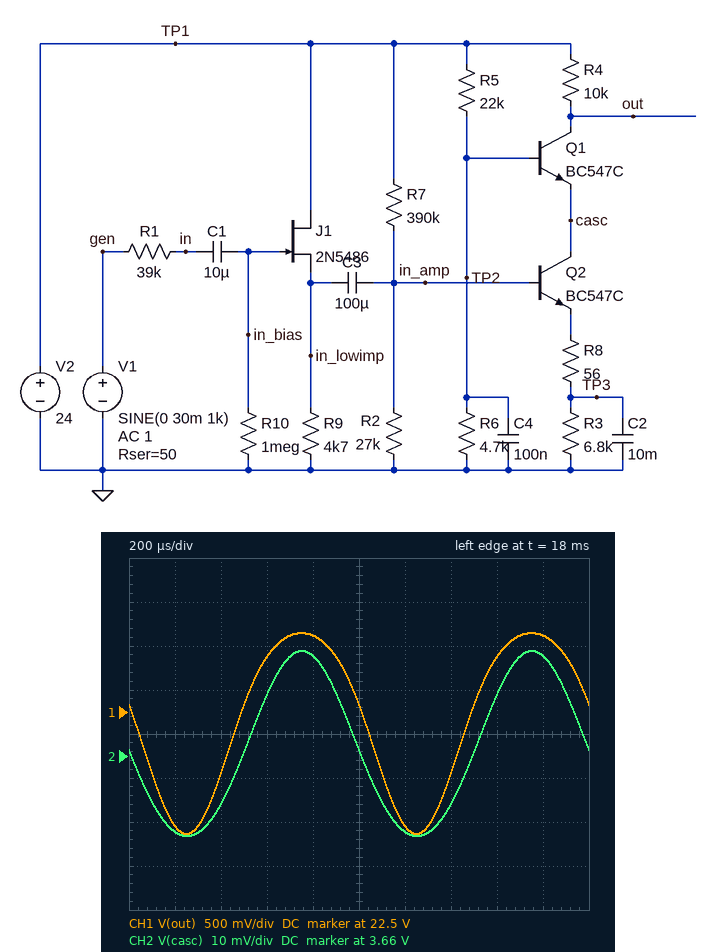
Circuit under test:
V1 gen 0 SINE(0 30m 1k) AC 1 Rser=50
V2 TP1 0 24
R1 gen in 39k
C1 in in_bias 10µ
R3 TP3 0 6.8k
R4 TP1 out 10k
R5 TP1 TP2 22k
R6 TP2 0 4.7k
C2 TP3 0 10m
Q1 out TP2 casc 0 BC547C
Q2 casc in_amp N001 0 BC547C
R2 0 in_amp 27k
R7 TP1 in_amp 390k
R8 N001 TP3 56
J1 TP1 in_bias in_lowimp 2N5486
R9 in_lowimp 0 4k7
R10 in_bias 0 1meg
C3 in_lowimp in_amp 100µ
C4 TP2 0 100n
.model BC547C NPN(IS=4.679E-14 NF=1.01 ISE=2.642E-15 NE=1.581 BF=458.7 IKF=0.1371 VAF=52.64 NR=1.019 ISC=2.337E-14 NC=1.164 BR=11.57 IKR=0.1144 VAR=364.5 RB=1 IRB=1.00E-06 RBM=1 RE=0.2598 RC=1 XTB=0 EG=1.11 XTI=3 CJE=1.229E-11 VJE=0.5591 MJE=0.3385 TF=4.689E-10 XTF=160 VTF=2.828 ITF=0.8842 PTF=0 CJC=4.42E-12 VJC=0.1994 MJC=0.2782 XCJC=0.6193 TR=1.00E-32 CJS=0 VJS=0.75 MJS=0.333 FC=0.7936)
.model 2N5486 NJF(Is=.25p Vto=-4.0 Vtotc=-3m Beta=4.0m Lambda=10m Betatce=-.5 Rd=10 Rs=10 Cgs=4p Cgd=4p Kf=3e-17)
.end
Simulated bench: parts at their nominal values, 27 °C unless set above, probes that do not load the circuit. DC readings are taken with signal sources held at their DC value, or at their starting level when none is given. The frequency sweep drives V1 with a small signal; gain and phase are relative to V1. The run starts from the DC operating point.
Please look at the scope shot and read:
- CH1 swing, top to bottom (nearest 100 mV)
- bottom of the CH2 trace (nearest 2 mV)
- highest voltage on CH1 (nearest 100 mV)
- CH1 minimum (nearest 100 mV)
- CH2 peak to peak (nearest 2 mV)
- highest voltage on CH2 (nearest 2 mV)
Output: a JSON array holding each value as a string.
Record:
["2.3 V", "3.642 V", "23.4 V", "21.1 V", "42 mV", "3.684 V"]
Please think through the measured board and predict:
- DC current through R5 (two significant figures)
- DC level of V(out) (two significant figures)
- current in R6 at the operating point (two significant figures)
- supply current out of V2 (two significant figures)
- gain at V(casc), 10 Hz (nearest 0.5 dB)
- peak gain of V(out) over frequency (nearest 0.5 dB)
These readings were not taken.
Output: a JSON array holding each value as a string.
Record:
["900 µA", "23 V", "900 µA", "1.9 mA", "-3.0 dB", "31.5 dB"]
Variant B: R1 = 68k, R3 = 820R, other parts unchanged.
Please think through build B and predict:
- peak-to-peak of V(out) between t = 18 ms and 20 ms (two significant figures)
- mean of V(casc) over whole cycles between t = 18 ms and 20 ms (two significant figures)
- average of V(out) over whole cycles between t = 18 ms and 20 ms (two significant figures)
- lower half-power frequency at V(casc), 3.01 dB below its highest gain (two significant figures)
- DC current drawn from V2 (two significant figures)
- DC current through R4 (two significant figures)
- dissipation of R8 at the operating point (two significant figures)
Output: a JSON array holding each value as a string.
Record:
["6.3 V", "3.6 V", "14 V", "270 mHz", "2.7 mA", "1.0 mA", "56 µW"]
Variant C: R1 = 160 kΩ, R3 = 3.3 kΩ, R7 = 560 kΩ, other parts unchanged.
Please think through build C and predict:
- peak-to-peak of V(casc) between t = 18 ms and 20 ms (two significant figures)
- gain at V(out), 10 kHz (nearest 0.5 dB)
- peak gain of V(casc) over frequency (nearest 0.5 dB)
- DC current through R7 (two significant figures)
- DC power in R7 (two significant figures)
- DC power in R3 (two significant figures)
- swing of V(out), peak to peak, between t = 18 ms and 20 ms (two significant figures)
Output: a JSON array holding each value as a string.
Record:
["37 mV", "31.0 dB", "-4.0 dB", "41 µA", "940 µW", "80 µW", "2.2 V"]
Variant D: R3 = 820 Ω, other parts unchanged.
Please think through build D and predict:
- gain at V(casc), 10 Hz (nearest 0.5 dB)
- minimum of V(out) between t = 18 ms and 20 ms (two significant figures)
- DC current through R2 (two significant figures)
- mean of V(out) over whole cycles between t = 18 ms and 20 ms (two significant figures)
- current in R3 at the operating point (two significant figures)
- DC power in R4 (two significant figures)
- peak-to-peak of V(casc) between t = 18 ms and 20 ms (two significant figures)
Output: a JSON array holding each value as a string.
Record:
["-7.5 dB", "11 V", "56 µA", "14 V", "1.0 mA", "10 mW", "21 mV"]
